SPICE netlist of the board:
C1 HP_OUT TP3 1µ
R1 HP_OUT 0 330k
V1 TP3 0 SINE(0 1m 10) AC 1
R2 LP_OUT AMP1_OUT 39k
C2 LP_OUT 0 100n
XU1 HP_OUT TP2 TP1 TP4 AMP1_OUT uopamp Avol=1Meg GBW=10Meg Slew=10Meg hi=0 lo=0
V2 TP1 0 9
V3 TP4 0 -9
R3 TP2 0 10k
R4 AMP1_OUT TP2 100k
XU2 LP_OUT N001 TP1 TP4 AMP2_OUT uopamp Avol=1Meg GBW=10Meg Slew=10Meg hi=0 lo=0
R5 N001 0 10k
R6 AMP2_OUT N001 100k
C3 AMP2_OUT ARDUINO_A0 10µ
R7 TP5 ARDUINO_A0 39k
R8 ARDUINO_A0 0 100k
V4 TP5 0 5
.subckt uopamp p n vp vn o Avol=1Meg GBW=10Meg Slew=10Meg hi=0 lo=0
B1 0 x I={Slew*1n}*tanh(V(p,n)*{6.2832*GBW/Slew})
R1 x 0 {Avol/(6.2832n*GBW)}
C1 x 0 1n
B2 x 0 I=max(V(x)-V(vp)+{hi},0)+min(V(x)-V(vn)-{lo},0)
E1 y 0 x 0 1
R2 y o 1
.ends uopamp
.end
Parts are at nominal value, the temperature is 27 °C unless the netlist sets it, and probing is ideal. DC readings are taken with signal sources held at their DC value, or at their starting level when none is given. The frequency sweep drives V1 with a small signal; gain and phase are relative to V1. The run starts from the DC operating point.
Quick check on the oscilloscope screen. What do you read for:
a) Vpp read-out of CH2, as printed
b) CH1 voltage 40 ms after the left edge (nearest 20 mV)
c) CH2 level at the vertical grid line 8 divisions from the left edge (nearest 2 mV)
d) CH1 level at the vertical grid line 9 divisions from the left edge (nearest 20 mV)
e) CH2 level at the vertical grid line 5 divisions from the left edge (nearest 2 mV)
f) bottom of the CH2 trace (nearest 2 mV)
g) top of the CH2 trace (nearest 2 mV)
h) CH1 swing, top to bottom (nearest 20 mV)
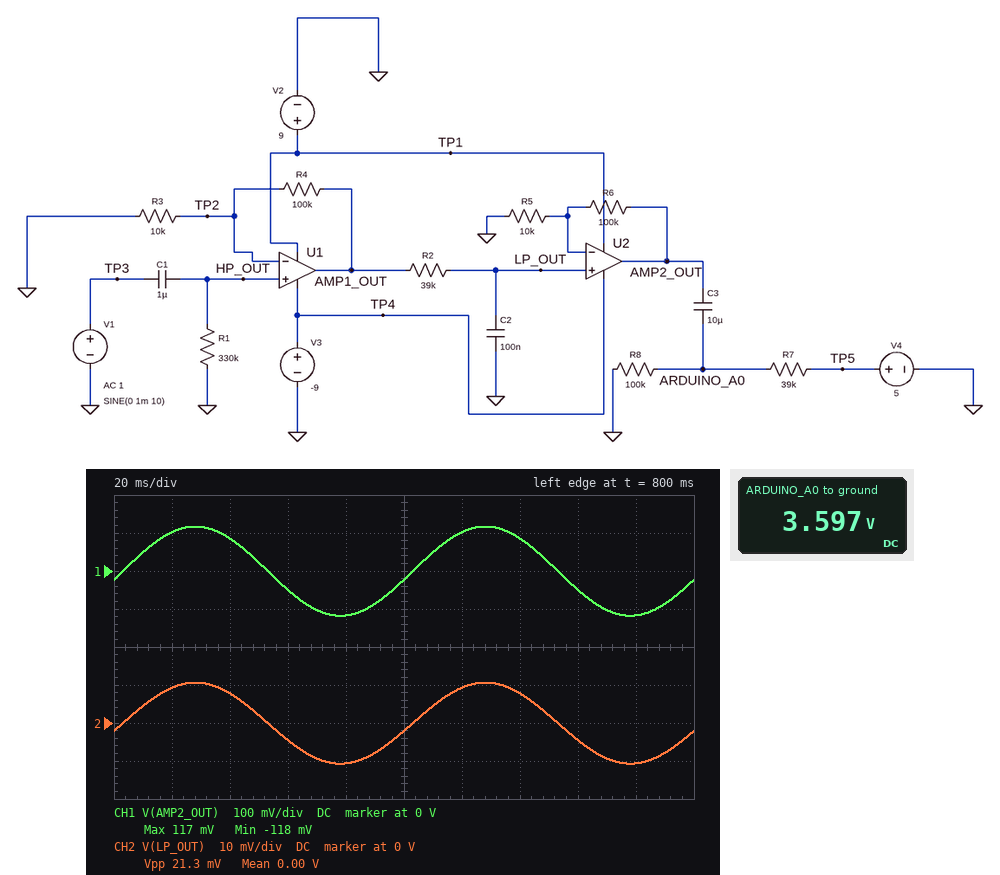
21.3 mV
80 mV
-4 mV
-120 mV
-2 mV
-10 mV
10 mV
240 mV
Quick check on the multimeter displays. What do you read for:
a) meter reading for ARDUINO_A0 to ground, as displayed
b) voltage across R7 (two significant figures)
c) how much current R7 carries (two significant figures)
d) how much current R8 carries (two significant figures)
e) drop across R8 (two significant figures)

3.597 V
1.4 V
36 µA
36 µA
3.6 V
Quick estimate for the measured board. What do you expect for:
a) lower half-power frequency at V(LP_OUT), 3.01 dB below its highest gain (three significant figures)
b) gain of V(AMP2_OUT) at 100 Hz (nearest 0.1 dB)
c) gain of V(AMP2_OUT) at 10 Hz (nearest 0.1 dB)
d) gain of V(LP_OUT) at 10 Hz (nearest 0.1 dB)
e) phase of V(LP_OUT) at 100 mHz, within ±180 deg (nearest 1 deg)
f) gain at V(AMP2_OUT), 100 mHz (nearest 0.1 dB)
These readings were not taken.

471 mHz
33.2 dB
41.4 dB
20.6 dB
78 deg
27.8 dB
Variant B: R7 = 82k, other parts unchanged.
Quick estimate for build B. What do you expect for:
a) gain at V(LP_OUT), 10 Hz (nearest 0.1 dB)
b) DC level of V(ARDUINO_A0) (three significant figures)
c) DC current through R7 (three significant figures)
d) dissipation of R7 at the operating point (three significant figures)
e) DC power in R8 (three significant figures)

20.6 dB
2.75 V
27.5 µA
61.9 µW
75.5 µW
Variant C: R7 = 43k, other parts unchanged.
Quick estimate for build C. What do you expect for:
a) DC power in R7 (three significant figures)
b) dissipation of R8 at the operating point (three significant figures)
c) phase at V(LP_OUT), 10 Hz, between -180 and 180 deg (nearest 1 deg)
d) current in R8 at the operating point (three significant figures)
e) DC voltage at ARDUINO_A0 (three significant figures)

52.6 µW
122 µW
-11 deg
35.0 µA
3.50 V
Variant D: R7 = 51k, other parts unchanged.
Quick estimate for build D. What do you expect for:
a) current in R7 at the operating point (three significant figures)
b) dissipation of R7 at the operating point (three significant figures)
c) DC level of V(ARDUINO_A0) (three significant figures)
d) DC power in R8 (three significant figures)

33.1 µA
55.9 µW
3.31 V
110 µW
